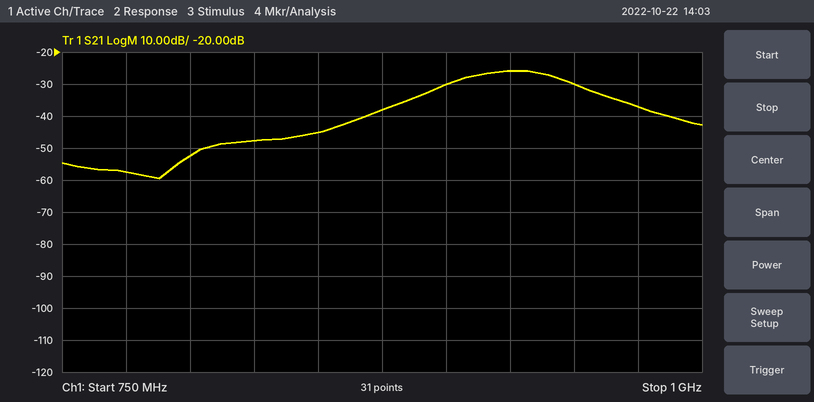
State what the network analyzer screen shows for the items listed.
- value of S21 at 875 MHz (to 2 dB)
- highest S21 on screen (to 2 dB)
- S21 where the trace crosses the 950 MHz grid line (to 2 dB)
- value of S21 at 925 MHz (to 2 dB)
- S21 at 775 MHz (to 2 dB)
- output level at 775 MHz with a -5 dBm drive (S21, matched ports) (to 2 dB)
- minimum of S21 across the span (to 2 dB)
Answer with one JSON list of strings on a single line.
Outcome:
["-38 dB", "-26 dB", "-30 dB", "-26 dB", "-58 dB", "-62 dBm", "-60 dB"]
